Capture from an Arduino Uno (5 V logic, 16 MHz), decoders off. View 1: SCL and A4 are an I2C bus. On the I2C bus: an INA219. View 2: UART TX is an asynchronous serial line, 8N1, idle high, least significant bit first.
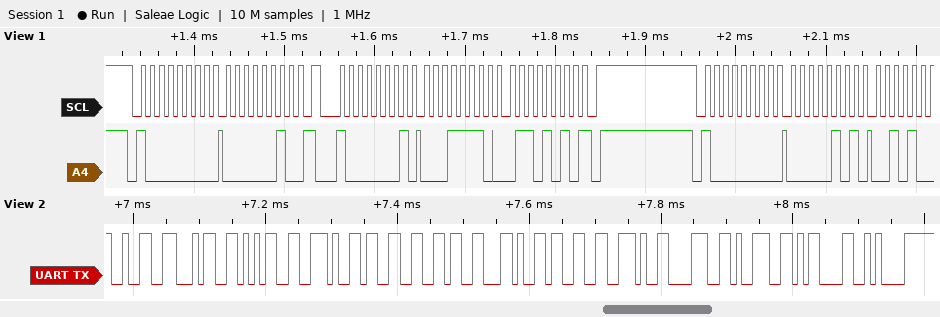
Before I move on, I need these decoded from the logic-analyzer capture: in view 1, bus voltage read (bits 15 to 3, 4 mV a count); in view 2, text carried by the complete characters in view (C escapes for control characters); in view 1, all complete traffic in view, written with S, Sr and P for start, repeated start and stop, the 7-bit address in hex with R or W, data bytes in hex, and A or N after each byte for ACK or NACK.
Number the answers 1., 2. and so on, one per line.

1. 3.892 V
2. "245.36,3.89\r\n"
3. S 40W A 02 A Sr 40R A 1E A 6A N P S 40W A 05 A
